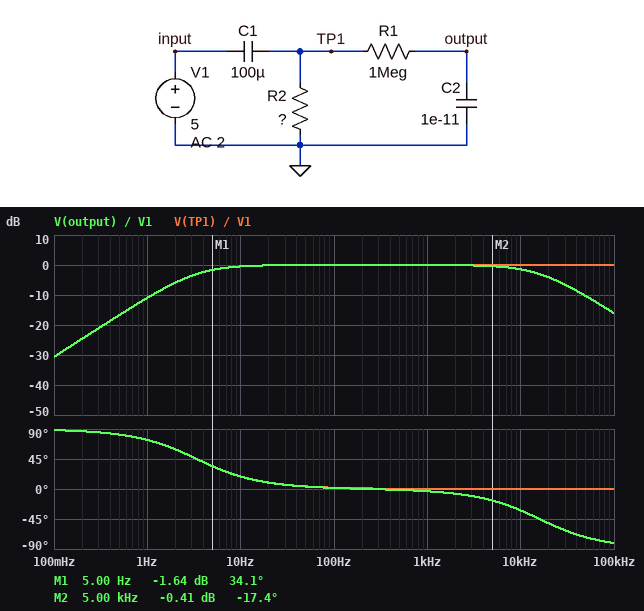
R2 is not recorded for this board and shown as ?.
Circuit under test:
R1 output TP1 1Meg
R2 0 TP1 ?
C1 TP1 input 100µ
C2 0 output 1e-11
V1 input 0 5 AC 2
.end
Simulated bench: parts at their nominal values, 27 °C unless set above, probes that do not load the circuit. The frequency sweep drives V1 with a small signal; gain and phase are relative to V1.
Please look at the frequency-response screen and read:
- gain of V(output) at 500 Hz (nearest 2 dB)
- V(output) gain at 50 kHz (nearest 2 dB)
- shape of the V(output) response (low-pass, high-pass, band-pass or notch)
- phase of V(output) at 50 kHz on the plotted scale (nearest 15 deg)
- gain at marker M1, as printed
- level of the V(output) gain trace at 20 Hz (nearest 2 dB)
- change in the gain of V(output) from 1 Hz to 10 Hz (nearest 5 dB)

0 dB
-10 dB
band-pass
-75 deg
-1.64 dB
0 dB
10 dB
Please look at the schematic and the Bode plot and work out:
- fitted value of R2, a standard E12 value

470 Ω
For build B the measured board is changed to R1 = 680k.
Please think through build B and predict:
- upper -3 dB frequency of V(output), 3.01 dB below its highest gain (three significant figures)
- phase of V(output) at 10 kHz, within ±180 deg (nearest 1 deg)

23.4 kHz
-23 deg
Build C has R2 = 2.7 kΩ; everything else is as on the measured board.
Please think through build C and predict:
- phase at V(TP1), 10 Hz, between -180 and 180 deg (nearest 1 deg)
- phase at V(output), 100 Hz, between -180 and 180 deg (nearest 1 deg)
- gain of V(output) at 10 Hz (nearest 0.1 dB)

3 deg
0 deg
0 dB
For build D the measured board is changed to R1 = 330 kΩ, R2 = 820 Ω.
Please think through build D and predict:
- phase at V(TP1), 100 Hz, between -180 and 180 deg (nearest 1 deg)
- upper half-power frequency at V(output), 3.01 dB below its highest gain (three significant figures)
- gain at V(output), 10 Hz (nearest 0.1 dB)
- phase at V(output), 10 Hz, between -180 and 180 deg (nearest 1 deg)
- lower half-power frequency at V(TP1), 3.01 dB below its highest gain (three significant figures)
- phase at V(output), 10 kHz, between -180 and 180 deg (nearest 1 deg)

1 deg
48.2 kHz
-0.2 dB
11 deg
1.94 Hz
-12 deg
